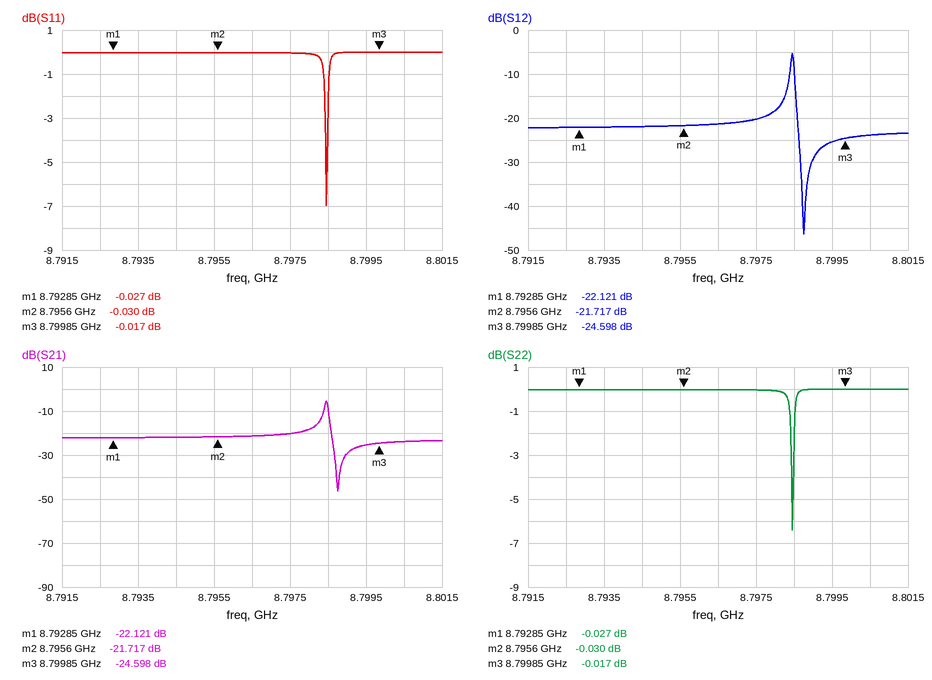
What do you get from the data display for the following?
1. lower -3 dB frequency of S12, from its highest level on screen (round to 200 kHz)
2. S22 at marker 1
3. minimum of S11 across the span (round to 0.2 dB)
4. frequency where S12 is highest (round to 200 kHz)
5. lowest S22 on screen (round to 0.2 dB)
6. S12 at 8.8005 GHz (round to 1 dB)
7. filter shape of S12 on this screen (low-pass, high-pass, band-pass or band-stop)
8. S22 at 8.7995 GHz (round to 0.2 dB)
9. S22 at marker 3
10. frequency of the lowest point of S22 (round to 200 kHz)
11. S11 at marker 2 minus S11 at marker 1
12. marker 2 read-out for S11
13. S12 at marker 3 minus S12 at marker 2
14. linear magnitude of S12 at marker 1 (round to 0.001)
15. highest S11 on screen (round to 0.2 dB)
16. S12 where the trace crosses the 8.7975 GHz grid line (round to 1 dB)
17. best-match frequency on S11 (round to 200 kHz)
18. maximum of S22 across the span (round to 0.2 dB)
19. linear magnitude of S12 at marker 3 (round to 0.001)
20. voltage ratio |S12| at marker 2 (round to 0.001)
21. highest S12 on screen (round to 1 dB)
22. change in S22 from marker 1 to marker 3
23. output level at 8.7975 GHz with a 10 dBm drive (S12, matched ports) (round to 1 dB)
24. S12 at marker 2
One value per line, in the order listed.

8.7984 GHz
-0.027 dB
-7.0 dB
8.7984 GHz
-6.4 dB
-24 dB
band-pass
0.0 dB
-0.017 dB
8.7984 GHz
-0.003 dB
-0.030 dB
-2.881 dB
0.078
0.0 dB
-20 dB
8.7984 GHz
0.0 dB
0.059
0.082
-5 dB
0.010 dB
-10 dBm
-21.717 dB
